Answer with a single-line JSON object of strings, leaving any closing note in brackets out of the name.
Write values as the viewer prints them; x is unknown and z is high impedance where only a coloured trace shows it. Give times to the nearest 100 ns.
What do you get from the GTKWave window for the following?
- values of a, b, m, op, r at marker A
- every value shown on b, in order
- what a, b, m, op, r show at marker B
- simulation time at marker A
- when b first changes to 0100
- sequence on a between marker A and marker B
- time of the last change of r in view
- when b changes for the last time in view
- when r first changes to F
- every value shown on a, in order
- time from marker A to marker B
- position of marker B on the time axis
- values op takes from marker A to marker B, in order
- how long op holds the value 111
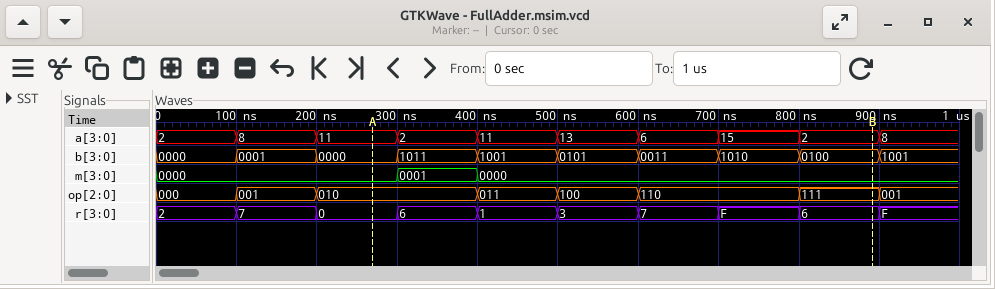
{"values of a, b, m, op, r at marker A": "a=11, b=0000, m=0000, op=010, r=0", "every value shown on b, in order": "0000, 0001, 0000, 1011, 1001, 0101, 0011, 1010, 0100, 1001", "what a, b, m, op, r show at marker B": "a=2, b=0100, m=0000, op=111, r=6", "simulation time at marker A": "300 ns", "when b first changes to 0100": "800 ns", "sequence on a between marker A and marker B": "11, 2, 11, 13, 6, 15, 2", "time of the last change of r in view": "900 ns", "when b changes for the last time in view": "900 ns", "when r first changes to F": "700 ns", "every value shown on a, in order": "2, 8, 11, 2, 11, 13, 6, 15, 2, 8", "time from marker A to marker B": "600 ns", "position of marker B on the time axis": "900 ns", "values op takes from marker A to marker B, in order": "010, 011, 100, 110, 111", "how long op holds the value 111": "100 ns"}
